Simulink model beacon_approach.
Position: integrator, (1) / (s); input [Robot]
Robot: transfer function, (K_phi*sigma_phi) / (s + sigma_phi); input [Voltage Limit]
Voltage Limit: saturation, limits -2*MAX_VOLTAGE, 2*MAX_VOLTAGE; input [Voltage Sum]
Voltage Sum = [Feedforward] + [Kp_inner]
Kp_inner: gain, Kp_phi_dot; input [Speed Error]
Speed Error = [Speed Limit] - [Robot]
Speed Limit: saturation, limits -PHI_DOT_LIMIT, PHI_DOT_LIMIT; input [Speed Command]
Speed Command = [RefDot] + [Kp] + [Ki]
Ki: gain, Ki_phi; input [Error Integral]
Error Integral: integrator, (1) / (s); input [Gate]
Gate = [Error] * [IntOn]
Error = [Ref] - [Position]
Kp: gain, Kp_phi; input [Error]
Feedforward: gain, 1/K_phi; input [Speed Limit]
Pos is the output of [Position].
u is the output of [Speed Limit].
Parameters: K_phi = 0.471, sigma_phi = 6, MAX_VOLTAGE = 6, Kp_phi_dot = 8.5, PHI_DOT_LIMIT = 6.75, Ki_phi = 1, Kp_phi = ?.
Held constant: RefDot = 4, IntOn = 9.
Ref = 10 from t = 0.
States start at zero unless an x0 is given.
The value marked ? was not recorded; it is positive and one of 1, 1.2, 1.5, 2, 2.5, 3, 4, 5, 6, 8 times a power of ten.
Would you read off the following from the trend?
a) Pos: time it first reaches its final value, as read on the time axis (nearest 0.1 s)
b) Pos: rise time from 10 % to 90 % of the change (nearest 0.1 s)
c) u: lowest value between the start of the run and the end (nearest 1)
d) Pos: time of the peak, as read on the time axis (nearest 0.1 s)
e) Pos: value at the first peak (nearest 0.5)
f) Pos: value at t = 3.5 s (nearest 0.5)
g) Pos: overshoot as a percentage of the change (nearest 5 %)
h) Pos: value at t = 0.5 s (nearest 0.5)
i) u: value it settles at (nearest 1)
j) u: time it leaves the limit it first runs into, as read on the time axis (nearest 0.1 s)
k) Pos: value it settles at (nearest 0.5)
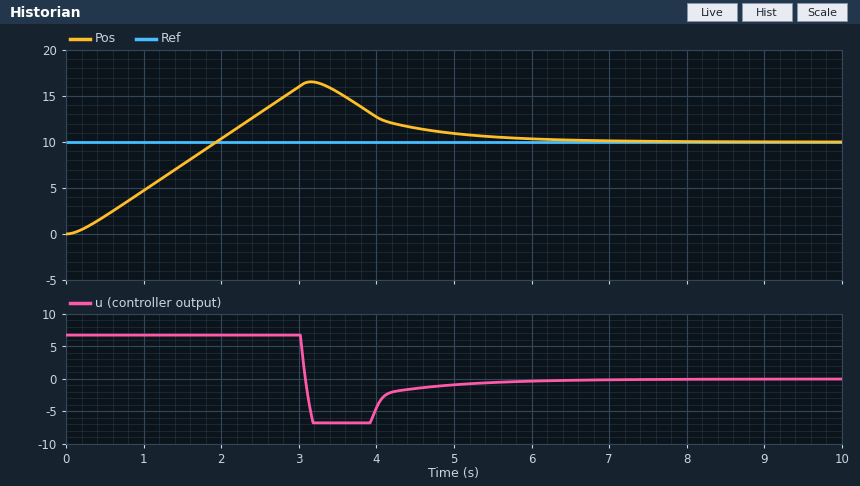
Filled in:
1.9 s
1.4 s
-7
3.2 s
16.5
15.5
65 %
2.0
0
3.0 s
10.0
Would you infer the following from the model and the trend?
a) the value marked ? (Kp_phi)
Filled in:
10
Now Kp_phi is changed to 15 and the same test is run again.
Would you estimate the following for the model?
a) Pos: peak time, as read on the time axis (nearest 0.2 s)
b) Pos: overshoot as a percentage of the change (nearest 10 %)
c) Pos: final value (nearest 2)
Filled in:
3.0 s
50 %
10
